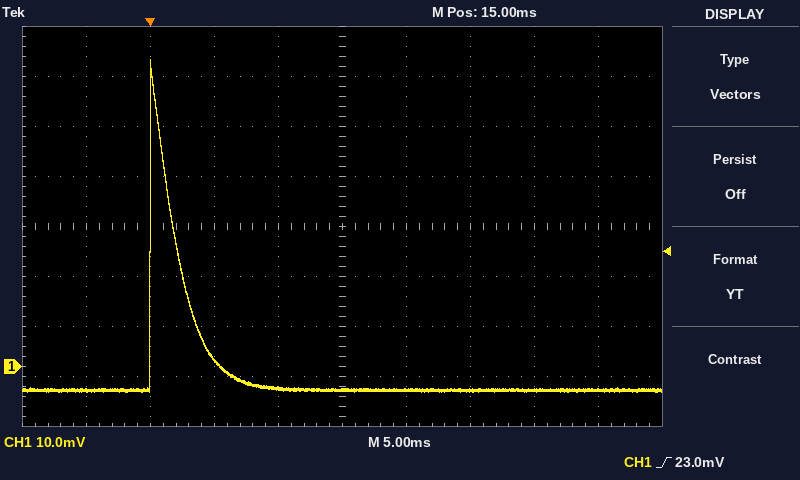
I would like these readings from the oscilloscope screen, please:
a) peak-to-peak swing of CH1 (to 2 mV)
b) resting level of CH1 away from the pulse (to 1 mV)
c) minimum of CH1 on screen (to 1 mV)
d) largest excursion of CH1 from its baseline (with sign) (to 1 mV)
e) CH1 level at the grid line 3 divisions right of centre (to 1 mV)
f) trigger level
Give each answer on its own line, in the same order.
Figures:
66 mV
-5 mV
-5 mV
+66 mV
-5 mV
23.0 mV
